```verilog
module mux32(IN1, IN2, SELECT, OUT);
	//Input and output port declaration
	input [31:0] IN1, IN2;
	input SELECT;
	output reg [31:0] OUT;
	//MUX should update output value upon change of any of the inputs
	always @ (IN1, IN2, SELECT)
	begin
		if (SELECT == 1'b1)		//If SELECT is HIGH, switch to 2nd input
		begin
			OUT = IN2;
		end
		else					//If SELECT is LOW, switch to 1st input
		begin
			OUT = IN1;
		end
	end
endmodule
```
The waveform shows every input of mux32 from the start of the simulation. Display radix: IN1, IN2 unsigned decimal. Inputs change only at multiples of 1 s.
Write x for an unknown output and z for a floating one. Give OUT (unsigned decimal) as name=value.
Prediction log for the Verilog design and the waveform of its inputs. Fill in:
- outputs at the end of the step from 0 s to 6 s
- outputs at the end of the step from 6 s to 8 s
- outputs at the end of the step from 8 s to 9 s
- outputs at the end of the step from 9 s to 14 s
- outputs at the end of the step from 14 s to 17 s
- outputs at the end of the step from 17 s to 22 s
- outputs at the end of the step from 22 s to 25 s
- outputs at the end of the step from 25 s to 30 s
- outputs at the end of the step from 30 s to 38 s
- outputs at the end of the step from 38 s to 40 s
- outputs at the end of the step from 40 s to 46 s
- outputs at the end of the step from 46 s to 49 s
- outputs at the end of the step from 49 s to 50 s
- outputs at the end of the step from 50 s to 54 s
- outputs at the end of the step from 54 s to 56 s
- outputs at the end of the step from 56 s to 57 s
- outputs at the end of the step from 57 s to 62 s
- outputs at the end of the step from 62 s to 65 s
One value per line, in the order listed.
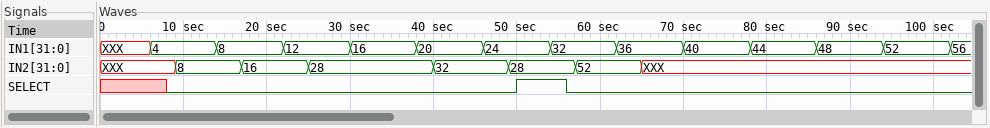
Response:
OUT=x
OUT=4
OUT=4
OUT=4
OUT=8
OUT=8
OUT=12
OUT=12
OUT=16
OUT=20
OUT=20
OUT=24
OUT=24
OUT=28
OUT=28
OUT=32
OUT=32
OUT=36
